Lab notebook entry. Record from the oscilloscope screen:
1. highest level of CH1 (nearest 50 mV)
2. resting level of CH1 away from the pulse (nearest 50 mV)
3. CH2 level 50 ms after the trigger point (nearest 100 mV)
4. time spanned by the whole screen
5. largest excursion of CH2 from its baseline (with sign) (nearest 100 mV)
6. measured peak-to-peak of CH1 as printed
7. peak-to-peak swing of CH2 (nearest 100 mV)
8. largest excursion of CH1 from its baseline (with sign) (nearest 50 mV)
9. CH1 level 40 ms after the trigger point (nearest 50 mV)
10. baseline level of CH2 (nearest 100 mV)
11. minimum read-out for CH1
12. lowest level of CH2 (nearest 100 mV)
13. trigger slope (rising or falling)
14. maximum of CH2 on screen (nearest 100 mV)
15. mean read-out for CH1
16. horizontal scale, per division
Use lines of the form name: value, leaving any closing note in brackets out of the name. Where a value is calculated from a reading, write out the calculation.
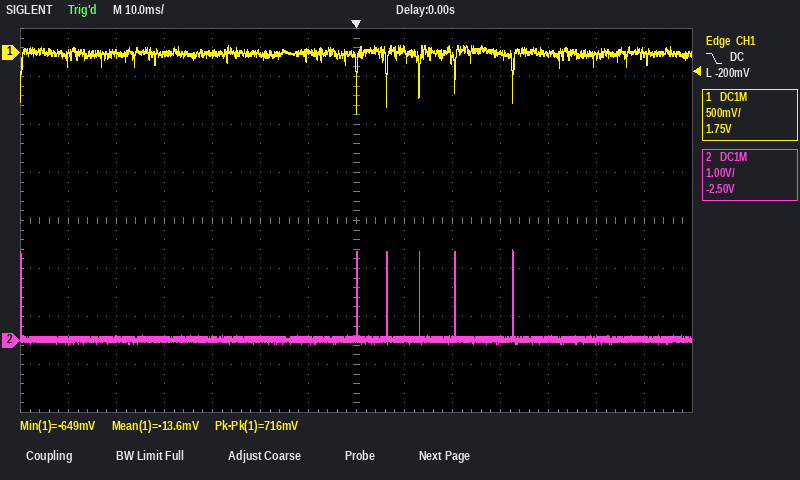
highest level of CH1: 50 mV
resting level of CH1 away from the pulse: 0 mV
CH2 level 50 ms after the trigger point: 0.0 V
time spanned by the whole screen: 140 ms
largest excursion of CH2 from its baseline (with sign): 1.9 V − (0.0 V) = +1.9 V
measured peak-to-peak of CH1 as printed: 716 mV
peak-to-peak swing of CH2: 1.9 V − (-100 mV) = 2.0 V
largest excursion of CH1 from its baseline (with sign): -650 mV
CH1 level 40 ms after the trigger point: 0 mV
baseline level of CH2: 0.0 V
minimum read-out for CH1: -649 mV
lowest level of CH2: -100 mV
trigger slope: falling
maximum of CH2 on screen: 1.9 V
mean read-out for CH1: -13.6 mV
horizontal scale, per division: 10 ms
